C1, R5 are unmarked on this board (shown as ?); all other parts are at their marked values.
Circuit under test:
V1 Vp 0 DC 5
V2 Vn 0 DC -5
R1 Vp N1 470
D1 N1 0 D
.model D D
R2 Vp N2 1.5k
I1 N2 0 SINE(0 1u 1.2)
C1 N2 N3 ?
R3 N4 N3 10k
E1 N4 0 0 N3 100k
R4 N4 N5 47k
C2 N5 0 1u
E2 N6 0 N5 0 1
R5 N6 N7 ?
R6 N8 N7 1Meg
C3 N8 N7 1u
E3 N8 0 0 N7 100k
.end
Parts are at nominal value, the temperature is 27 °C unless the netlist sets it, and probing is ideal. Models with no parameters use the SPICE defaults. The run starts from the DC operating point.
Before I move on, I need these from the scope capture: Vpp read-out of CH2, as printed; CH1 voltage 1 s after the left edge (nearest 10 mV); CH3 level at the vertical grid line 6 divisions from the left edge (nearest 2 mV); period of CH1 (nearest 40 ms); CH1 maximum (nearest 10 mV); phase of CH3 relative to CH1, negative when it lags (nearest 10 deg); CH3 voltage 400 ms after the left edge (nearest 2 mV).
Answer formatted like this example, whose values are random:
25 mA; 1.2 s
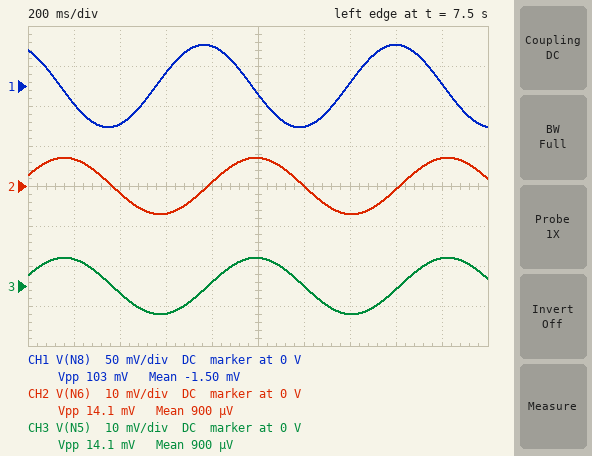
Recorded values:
14.1 mV; -10 mV; 0 V; 840 ms; 50 mV; -100 deg; -2 mV
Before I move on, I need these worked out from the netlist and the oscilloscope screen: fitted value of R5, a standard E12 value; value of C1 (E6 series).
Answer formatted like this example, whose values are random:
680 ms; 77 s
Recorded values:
18 kΩ; 100 µF
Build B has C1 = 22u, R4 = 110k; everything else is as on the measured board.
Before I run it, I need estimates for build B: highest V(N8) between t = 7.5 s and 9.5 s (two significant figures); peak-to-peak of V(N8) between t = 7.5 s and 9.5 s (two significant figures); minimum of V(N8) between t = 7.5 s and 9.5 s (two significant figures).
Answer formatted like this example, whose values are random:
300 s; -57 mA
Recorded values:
14 mV; 27 mV; -14 mV
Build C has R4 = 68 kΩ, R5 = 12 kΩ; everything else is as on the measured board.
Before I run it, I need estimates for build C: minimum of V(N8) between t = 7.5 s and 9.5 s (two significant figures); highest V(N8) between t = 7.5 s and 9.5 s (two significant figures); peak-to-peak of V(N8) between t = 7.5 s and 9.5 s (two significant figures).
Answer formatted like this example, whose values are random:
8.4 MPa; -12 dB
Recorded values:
-73 mV; 73 mV; 150 mV
